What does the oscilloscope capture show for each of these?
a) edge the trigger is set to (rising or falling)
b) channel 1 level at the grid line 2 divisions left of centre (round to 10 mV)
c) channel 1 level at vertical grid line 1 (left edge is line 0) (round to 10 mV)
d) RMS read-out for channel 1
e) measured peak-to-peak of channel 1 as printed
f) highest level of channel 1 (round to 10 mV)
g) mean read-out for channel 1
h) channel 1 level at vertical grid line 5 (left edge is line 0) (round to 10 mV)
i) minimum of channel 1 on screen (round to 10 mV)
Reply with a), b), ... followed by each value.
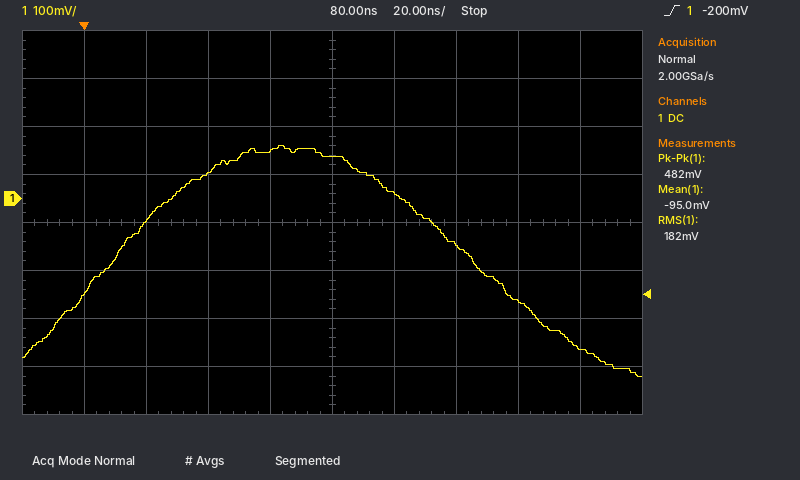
a) rising
b) 50 mV
c) -200 mV
d) 182 mV
e) 482 mV
f) 110 mV
g) -95.0 mV
h) 90 mV
i) -370 mV
